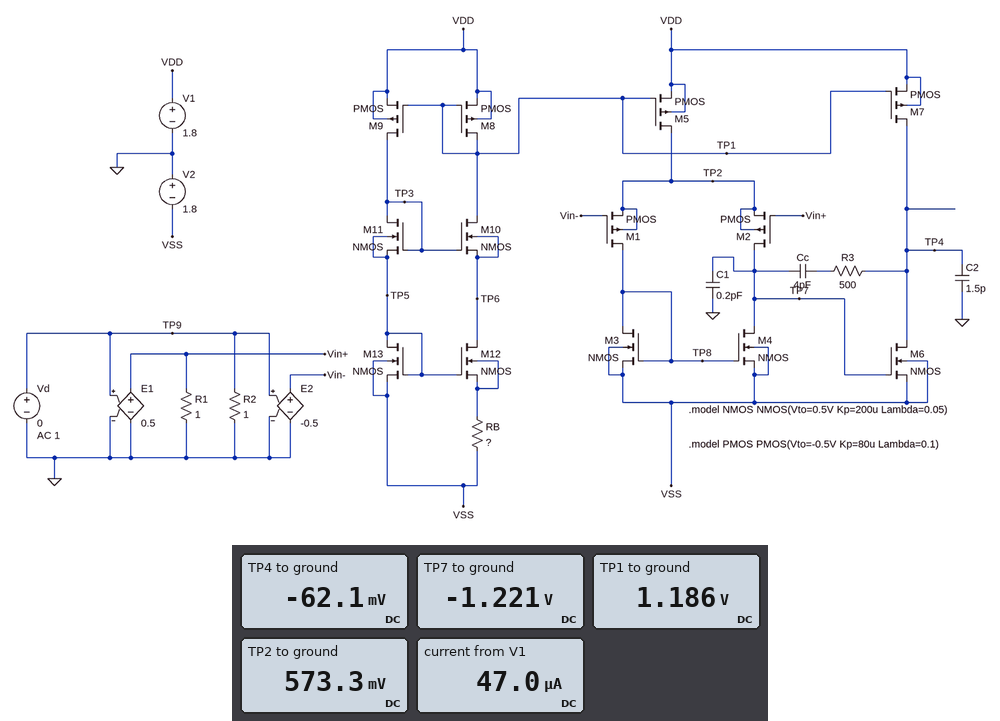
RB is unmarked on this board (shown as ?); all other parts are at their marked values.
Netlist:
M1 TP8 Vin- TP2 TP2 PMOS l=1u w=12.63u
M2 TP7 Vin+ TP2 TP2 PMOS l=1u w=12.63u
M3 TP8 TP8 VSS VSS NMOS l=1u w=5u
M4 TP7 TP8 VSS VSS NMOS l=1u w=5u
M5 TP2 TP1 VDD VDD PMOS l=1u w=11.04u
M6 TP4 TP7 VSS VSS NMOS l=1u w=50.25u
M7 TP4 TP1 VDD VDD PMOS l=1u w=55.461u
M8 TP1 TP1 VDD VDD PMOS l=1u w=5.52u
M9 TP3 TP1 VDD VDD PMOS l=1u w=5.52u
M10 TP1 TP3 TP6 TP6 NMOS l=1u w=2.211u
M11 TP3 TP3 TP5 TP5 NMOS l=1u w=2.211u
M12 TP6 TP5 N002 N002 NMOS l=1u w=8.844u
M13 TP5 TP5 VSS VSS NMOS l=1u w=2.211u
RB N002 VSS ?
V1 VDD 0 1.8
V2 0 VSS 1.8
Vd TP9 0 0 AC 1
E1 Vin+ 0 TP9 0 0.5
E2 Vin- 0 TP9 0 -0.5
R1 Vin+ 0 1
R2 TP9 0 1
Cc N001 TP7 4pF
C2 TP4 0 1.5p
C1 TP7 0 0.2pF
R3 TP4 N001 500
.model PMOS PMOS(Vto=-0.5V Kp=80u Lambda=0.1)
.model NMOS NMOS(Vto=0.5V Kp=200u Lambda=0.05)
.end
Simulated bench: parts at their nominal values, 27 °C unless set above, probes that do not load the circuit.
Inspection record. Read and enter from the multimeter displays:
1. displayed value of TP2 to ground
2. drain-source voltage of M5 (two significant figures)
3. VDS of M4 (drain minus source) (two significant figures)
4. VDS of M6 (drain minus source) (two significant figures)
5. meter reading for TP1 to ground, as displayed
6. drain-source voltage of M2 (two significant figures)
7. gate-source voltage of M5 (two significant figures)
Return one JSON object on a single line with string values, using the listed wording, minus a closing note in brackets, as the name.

{"displayed value of TP2 to ground": "573.3 mV", "drain-source voltage of M5": "-1.2 V", "VDS of M4 (drain minus source)": "580 mV", "VDS of M6 (drain minus source)": "1.7 V", "meter reading for TP1 to ground, as displayed": "1.186 V", "drain-source voltage of M2": "-1.8 V", "gate-source voltage of M5": "-610 mV"}
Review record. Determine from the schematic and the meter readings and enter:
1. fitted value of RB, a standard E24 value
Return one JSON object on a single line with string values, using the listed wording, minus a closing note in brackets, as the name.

{"fitted value of RB, a standard E24 value": "22 kΩ"}
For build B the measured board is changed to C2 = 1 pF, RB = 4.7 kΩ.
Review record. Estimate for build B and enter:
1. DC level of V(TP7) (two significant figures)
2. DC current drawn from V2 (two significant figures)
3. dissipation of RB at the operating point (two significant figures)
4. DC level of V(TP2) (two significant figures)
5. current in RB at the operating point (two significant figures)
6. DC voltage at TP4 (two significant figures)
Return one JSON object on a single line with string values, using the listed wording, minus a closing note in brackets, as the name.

{"DC level of V(TP7)": "-980 mV", "DC current drawn from V2": "790 µA", "dissipation of RB at the operating point": "14 µW", "DC level of V(TP2)": "800 mV", "current in RB at the operating point": "54 µA", "DC voltage at TP4": "180 mV"}
